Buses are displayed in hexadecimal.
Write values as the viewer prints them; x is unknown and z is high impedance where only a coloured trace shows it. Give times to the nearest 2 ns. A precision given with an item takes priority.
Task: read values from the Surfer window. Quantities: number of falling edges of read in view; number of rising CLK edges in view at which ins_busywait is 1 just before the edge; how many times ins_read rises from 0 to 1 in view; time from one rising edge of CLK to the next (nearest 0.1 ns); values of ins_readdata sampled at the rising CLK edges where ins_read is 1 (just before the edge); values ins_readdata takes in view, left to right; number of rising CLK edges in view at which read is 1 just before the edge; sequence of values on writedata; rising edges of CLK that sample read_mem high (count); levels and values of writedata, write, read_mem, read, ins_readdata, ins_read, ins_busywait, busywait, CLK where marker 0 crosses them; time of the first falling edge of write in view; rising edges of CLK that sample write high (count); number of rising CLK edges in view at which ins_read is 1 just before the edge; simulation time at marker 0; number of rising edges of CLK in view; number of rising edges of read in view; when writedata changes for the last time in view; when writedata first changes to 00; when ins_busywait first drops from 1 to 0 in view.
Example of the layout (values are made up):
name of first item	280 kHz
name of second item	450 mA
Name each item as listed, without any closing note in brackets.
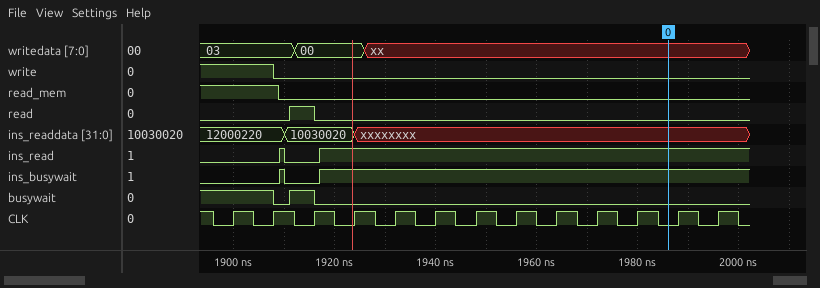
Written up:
number of falling edges of read in view	1
number of rising CLK edges in view at which ins_busywait is 1 just before the edge	10
how many times ins_read rises from 0 to 1 in view	2
time from one rising edge of CLK to the next	8 ns
values of ins_readdata sampled at the rising CLK edges where ins_read is 1	10030020, xxxxxxxx, xxxxxxxx, xxxxxxxx, xxxxxxxx, xxxxxxxx, xxxxxxxx, xxxxxxxx, xxxxxxxx, xxxxxxxx
values ins_readdata takes in view, left to right	12000220, 10030020, xxxxxxxx
number of rising CLK edges in view at which read is 1 just before the edge	1
sequence of values on writedata	03, 00, xx
rising edges of CLK that sample read_mem high	2
levels and values of writedata, write, read_mem, read, ins_readdata, ins_read, ins_busywait, busywait, CLK where marker 0 crosses them	writedata=xx, write=0, read_mem=0, read=0, ins_readdata=xxxxxxxx, ins_read=1, ins_busywait=1, busywait=0, CLK=0
time of the first falling edge of write in view	1908 ns
rising edges of CLK that sample write high	2
number of rising CLK edges in view at which ins_read is 1 just before the edge	10
simulation time at marker 0	1986 ns
number of rising edges of CLK in view	13
number of rising edges of read in view	1
when writedata changes for the last time in view	1926 ns
when writedata first changes to 00	1912 ns
when ins_busywait first drops from 1 to 0 in view	1910 ns
